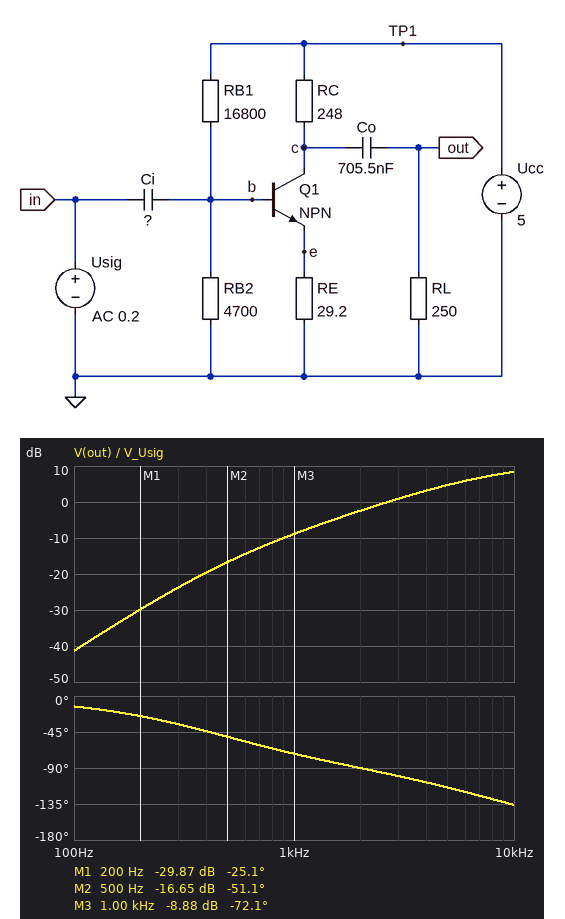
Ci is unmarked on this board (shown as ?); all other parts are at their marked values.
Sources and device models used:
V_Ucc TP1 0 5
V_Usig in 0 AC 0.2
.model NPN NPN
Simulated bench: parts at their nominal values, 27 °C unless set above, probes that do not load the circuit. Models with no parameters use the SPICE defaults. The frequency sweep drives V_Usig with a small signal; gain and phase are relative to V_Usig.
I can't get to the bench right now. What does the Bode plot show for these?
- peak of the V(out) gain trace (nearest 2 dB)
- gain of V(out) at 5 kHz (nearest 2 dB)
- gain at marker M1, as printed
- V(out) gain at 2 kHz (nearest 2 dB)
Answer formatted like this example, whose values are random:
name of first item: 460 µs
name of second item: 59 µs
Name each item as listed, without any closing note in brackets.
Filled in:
peak of the V(out) gain trace: 8 dB
gain of V(out) at 5 kHz: 4 dB
gain at marker M1, as printed: -29.87 dB
V(out) gain at 2 kHz: -2 dB
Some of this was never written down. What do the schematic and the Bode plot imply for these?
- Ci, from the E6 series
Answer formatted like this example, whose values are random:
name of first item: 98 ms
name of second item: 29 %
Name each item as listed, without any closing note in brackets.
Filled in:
Ci, from the E6 series: 10 nF
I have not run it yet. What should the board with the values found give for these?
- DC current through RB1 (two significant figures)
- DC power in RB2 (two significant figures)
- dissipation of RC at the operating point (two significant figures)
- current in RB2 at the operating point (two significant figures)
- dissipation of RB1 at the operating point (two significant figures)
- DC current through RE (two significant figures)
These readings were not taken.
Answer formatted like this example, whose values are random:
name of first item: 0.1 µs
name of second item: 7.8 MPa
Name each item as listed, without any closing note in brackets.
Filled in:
DC current through RB1: 240 µA
DC power in RB2: 190 µW
dissipation of RC at the operating point: 4.5 mW
current in RB2 at the operating point: 200 µA
dissipation of RB1 at the operating point: 980 µW
DC current through RE: 4.3 mA
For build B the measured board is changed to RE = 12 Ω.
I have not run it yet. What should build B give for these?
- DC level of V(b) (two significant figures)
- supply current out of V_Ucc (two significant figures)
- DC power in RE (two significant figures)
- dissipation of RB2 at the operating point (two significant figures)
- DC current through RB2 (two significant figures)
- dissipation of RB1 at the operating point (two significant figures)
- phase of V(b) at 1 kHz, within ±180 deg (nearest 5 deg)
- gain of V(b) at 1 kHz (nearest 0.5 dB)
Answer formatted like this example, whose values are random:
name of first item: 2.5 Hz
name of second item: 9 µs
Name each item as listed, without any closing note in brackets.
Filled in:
DC level of V(b): 890 mV
supply current out of V_Ucc: 5.9 mA
DC power in RE: 390 µW
dissipation of RB2 at the operating point: 170 µW
DC current through RB2: 190 µA
dissipation of RB1 at the operating point: 1.0 mW
phase of V(b) at 1 kHz, within ±180 deg: 85 deg
gain of V(b) at 1 kHz: -23.0 dB
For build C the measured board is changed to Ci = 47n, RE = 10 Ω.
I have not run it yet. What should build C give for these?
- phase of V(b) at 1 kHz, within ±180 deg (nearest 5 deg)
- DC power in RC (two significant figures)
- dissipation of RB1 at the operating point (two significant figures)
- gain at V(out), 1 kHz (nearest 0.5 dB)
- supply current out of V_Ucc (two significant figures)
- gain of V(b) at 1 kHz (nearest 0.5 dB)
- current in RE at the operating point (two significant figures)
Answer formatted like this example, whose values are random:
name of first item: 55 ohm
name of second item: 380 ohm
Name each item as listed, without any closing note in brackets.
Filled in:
phase of V(b) at 1 kHz, within ±180 deg: 75 deg
DC power in RC: 8.4 mW
dissipation of RB1 at the operating point: 1.0 mW
gain at V(out), 1 kHz: 7.0 dB
supply current out of V_Ucc: 6.1 mA
gain of V(b) at 1 kHz: -10.5 dB
current in RE at the operating point: 5.9 mA
